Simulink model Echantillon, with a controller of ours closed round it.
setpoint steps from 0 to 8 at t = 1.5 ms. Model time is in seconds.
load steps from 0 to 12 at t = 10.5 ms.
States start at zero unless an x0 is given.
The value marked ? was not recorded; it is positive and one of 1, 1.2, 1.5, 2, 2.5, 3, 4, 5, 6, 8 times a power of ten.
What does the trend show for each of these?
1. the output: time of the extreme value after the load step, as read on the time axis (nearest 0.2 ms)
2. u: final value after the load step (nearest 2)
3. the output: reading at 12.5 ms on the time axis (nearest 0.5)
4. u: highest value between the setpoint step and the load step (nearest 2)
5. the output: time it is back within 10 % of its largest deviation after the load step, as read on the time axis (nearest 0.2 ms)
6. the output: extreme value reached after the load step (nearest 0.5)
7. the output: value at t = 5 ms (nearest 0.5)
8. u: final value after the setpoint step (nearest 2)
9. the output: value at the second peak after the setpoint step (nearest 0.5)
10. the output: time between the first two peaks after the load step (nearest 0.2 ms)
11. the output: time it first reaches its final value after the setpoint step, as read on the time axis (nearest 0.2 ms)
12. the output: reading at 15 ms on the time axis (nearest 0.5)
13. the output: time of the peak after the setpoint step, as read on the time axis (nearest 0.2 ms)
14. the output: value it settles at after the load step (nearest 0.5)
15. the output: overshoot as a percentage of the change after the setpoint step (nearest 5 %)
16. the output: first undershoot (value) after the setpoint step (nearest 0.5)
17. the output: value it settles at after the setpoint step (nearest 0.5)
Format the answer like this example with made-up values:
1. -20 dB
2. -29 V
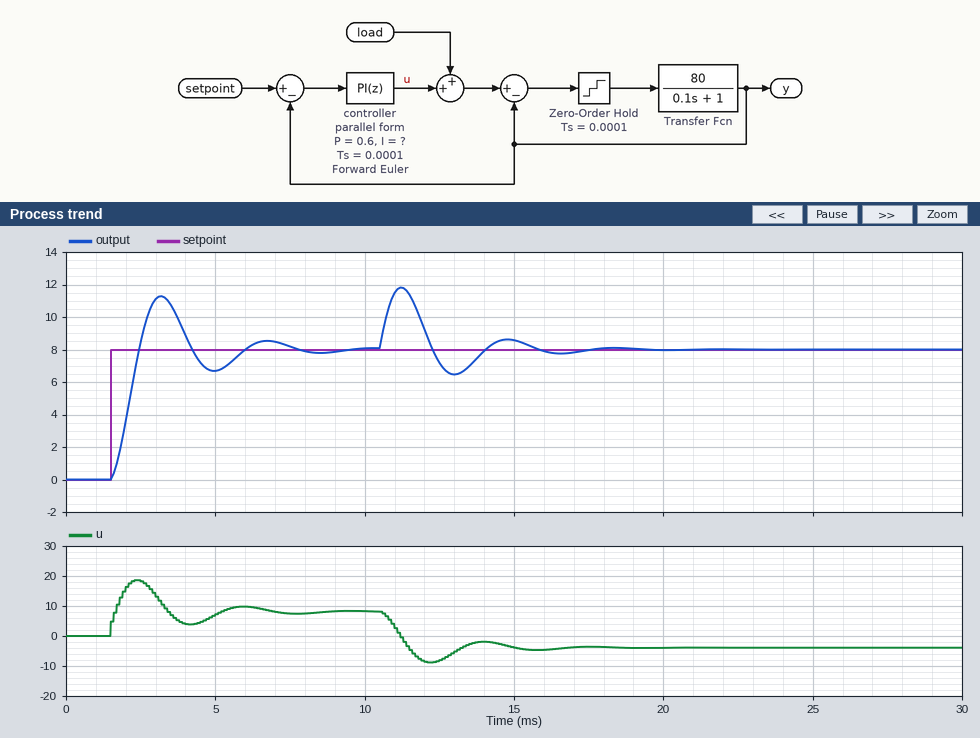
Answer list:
1. 11.2 ms
2. -4
3. 7.0
4. 18
5. 15.4 ms
6. 12.0
7. 6.5
8. 8
9. 8.5
10. 3.6 ms
11. 2.4 ms
12. 8.5
13. 3.2 ms
14. 8.0
15. 40 %
16. 6.5
17. 8.0
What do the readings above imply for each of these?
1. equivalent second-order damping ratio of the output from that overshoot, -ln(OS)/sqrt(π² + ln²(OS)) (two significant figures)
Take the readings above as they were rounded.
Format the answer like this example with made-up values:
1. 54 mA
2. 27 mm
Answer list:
1. 0.28
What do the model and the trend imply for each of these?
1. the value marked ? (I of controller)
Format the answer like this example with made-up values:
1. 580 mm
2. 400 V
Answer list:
1. 4000
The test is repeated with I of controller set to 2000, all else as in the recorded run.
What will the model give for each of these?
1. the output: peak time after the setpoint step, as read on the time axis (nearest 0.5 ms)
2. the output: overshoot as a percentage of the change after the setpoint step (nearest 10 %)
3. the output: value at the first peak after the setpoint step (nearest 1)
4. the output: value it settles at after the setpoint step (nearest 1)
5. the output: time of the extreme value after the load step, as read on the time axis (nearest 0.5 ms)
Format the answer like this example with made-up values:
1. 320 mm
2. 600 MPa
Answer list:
1. 4.0 ms
2. 20 %
3. 10
4. 8
5. 11.5 ms
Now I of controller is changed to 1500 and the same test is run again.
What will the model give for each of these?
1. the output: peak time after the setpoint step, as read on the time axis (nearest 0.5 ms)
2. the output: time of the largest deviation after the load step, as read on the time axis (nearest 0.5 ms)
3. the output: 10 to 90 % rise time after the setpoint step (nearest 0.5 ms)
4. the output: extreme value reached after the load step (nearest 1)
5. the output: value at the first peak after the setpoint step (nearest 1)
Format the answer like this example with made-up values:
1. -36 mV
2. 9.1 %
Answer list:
1. 4.5 ms
2. 11.5 ms
3. 1.5 ms
4. 13
5. 9
